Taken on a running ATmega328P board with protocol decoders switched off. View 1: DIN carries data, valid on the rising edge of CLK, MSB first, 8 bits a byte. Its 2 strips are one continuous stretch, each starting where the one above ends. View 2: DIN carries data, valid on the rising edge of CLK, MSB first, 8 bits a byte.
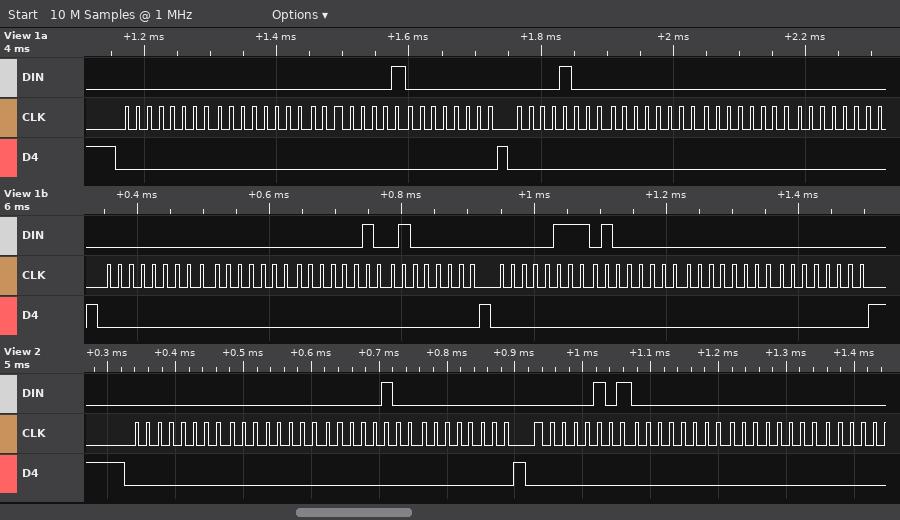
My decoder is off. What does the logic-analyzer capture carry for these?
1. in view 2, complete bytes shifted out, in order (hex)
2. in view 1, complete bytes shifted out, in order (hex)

00 00 04 00 05 00 00
00 00 01 00 08 00 00 00 00 00 02 40 07 40 00 00
